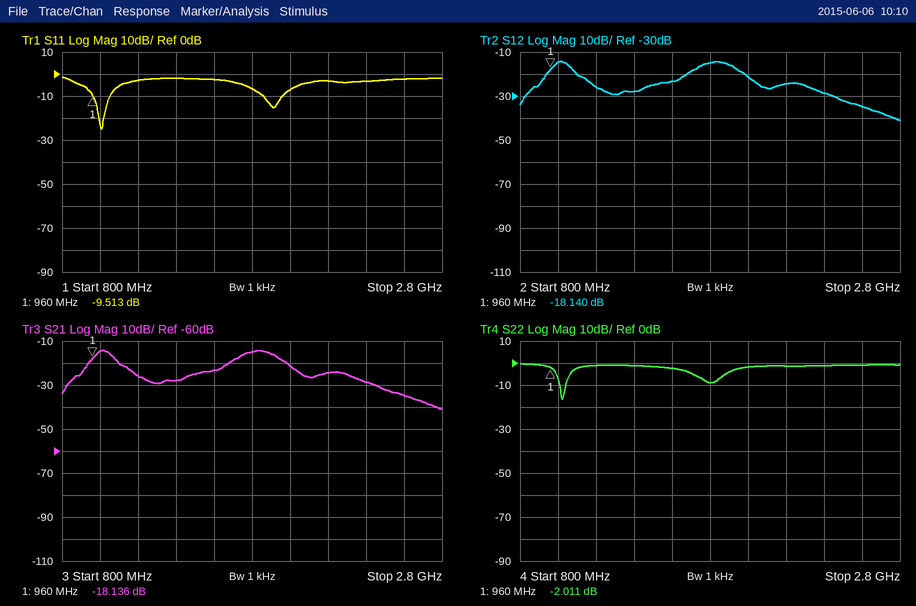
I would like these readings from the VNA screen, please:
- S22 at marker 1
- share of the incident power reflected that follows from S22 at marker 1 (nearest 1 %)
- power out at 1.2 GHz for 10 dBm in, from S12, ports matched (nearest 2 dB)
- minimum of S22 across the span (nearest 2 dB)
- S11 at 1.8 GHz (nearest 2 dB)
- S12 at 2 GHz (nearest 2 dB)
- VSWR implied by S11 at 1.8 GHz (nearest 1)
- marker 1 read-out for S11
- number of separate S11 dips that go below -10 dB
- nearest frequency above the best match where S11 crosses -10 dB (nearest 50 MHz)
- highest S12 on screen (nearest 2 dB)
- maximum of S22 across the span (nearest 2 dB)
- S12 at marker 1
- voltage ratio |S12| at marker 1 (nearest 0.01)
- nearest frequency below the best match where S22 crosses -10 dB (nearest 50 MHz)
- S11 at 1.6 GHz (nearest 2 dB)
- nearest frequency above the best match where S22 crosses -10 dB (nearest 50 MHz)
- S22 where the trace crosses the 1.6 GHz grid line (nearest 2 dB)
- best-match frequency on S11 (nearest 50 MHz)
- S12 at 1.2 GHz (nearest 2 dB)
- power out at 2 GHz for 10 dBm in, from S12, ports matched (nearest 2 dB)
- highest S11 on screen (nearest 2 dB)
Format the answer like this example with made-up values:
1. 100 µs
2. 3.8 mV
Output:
1. -2.011 dB
2. 63 %
3. -16 dBm
4. -16 dB
5. -6 dB
6. -22 dB
7. 3
8. -9.513 dB
9. 2
10. 1.05 GHz
11. -14 dB
12. 0 dB
13. -18.140 dB
14. 0.12
15. 1.00 GHz
16. -2 dB
17. 1.05 GHz
18. -2 dB
19. 1.00 GHz
20. -26 dB
21. -12 dBm
22. -2 dB
